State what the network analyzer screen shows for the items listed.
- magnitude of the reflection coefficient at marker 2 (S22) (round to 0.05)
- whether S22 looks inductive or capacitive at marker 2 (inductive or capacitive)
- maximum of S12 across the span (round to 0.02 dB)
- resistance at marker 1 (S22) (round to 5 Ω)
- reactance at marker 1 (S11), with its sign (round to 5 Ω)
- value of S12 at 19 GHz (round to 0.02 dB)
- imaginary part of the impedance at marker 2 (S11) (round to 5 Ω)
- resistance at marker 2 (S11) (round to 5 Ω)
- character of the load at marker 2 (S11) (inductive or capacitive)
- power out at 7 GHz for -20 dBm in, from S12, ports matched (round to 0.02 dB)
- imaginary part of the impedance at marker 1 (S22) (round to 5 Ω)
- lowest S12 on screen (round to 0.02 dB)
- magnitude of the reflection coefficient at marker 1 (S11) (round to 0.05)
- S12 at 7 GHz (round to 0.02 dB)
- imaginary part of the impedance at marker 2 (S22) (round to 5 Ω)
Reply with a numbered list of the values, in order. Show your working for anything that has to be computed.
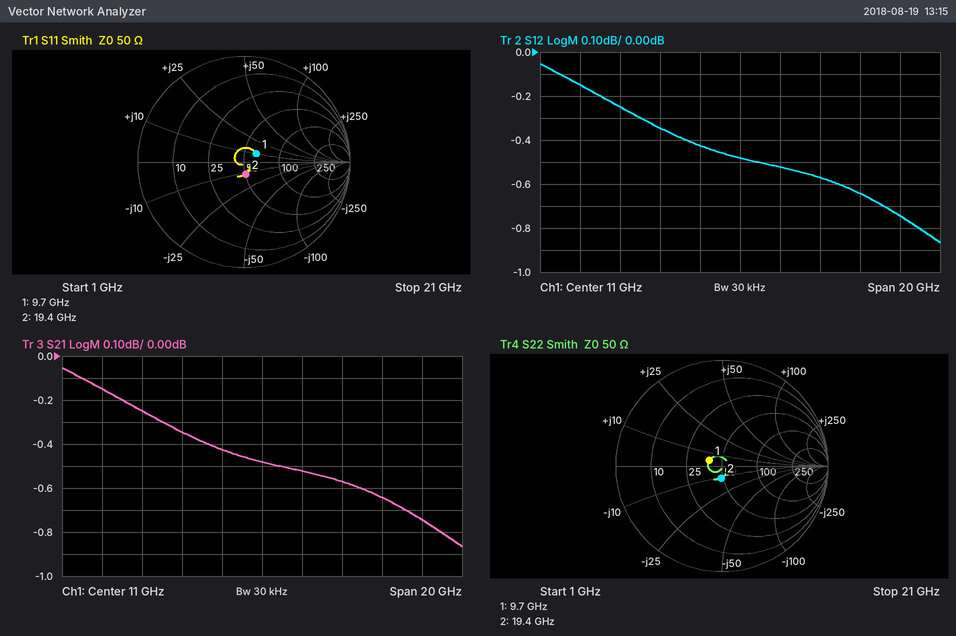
1. 0.10
2. capacitive
3. -0.06 dB
4. 40 Ω
5. +10 Ω
6. -0.74 dB
7. -10 Ω
8. 50 Ω
9. capacitive
10. -20 dBm + (-0.34 dB) = -20.34 dBm
11. +5 Ω
12. -0.86 dB
13. 0.15
14. -0.34 dB
15. -10 Ω
